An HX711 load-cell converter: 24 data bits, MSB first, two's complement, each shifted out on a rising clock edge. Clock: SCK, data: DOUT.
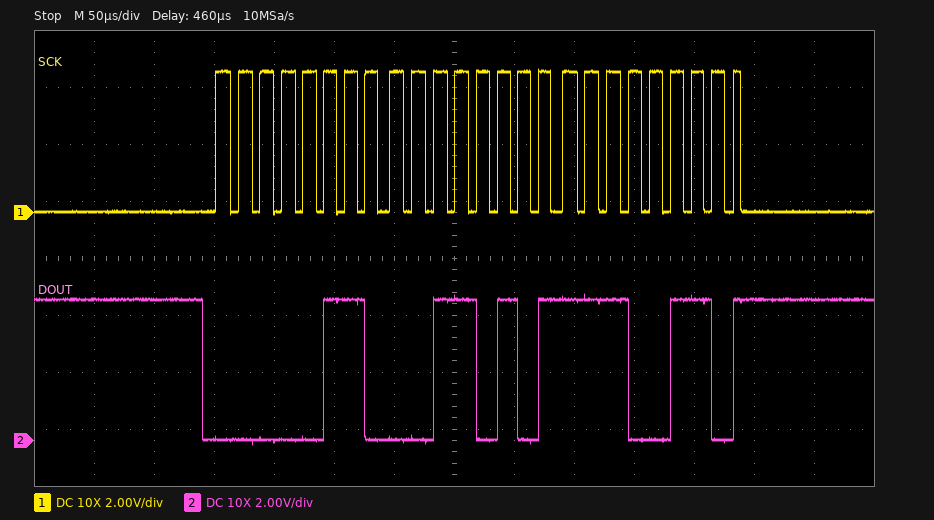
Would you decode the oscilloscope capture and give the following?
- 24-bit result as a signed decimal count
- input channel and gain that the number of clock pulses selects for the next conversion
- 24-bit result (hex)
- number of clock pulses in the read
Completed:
407014
channel A, gain 128
0x0635E6
25
